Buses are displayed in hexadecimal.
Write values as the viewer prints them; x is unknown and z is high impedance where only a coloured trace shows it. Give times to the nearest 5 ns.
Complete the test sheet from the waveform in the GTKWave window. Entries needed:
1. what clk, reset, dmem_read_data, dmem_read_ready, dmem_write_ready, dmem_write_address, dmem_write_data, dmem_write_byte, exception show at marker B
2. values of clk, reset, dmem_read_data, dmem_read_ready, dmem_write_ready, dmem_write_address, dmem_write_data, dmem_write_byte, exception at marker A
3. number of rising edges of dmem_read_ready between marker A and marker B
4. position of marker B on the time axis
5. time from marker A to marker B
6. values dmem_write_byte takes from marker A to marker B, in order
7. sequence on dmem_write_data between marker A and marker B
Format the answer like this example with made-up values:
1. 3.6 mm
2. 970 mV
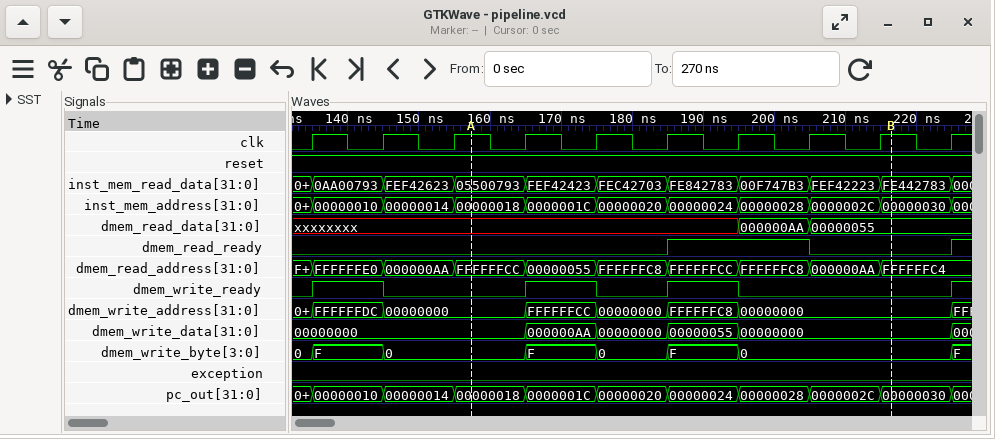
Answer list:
1. clk=1, reset=1, dmem_read_data=00000055, dmem_read_ready=0, dmem_write_ready=0, dmem_write_address=00000000, dmem_write_data=00000000, dmem_write_byte=0, exception=0
2. clk=1, reset=1, dmem_read_data=xxxxxxxx, dmem_read_ready=0, dmem_write_ready=0, dmem_write_address=00000000, dmem_write_data=00000000, dmem_write_byte=0, exception=0
3. 1
4. 215 ns
5. 60 ns
6. 0, F, 0, F, 0
7. 00000000, 000000AA, 00000000, 00000055, 00000000
